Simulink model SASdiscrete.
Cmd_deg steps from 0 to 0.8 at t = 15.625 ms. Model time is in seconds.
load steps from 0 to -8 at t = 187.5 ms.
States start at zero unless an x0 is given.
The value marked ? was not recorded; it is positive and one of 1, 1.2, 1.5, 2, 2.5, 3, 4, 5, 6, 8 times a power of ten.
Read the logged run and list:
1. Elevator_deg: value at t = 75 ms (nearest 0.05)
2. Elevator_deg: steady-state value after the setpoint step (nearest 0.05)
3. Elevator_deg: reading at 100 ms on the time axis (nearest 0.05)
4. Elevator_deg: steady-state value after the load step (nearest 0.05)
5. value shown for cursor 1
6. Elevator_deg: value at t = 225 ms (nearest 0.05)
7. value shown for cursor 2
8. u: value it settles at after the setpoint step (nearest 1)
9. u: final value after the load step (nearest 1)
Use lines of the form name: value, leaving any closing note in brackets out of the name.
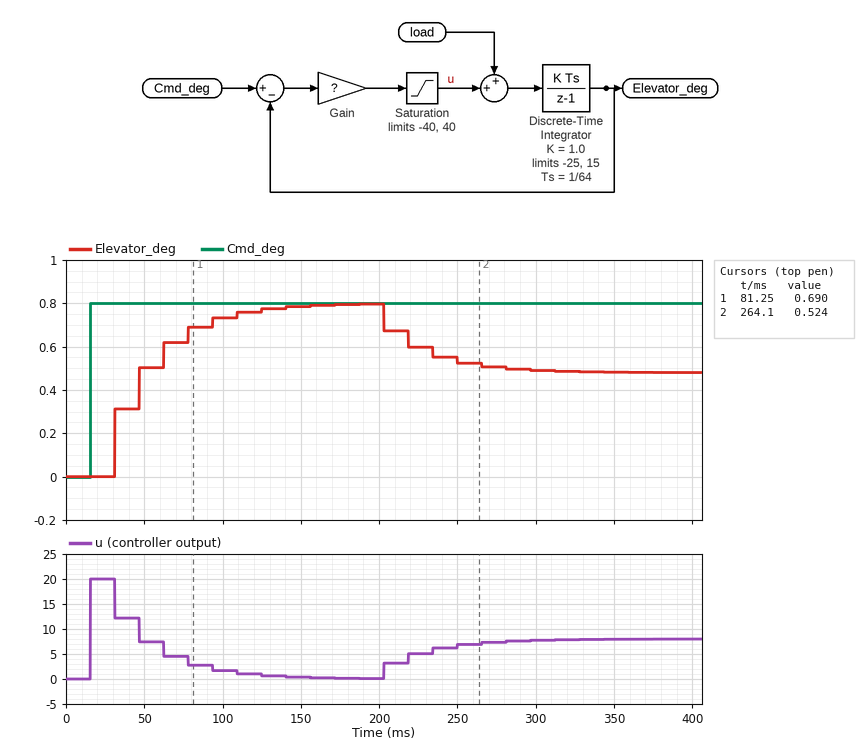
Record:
Elevator_deg: value at t = 75 ms: 0.60
Elevator_deg: steady-state value after the setpoint step: 0.80
Elevator_deg: reading at 100 ms on the time axis: 0.75
Elevator_deg: steady-state value after the load step: 0.50
value shown for cursor 1: 0.690
Elevator_deg: value at t = 225 ms: 0.60
value shown for cursor 2: 0.524
u: value it settles at after the setpoint step: 0
u: final value after the load step: 8
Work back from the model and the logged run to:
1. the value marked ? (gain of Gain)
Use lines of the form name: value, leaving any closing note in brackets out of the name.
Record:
the value marked ?: 25
